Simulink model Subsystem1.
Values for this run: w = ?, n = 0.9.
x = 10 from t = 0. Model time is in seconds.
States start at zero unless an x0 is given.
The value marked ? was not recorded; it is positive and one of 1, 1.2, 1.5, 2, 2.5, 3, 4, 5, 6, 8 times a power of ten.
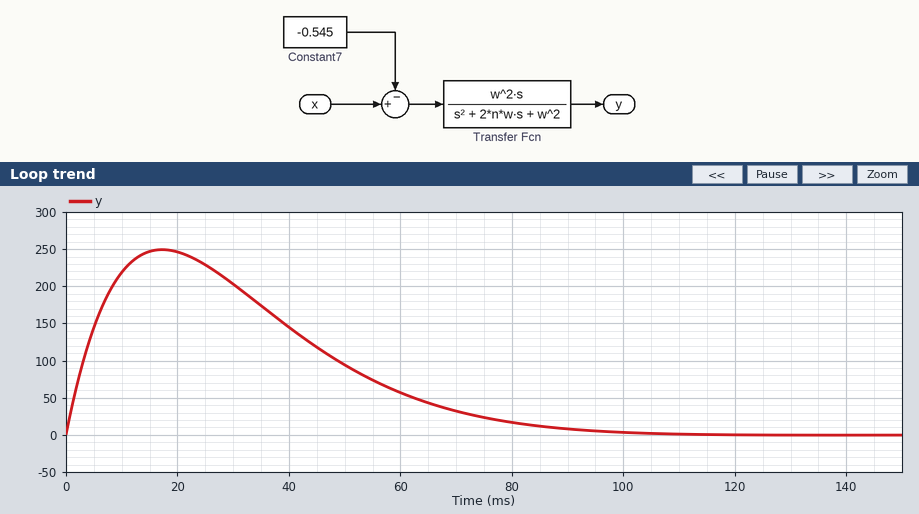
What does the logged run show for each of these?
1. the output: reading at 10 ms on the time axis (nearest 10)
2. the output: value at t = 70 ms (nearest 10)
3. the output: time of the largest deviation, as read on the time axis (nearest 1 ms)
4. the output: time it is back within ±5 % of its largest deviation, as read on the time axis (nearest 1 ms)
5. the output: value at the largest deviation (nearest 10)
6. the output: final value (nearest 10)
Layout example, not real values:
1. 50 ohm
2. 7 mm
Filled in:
1. 220
2. 30
3. 17 ms
4. 84 ms
5. 250
6. 0
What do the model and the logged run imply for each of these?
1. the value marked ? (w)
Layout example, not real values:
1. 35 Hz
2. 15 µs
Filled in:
1. 60
